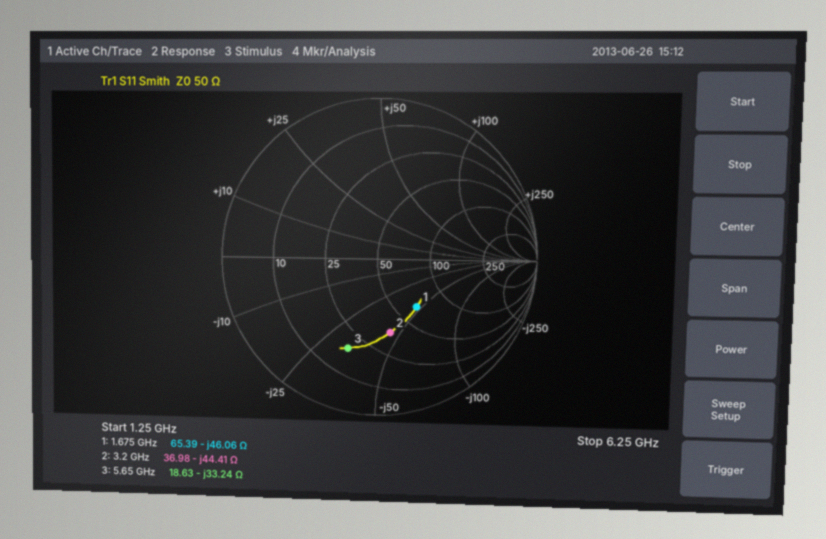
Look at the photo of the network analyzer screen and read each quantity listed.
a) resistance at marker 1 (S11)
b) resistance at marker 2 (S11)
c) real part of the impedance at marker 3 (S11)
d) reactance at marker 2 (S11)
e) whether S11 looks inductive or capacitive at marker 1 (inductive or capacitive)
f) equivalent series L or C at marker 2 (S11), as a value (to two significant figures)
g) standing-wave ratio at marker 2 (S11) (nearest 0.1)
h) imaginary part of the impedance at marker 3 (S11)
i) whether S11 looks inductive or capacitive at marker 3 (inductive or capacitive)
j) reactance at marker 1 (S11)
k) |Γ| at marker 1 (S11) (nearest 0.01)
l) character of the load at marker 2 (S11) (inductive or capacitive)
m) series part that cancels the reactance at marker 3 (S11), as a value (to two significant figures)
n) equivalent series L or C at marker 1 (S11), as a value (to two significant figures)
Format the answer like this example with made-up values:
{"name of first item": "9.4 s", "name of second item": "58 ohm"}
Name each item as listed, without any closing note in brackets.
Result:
{"resistance at marker 1": "65.39 Ω", "resistance at marker 2": "36.98 Ω", "real part of the impedance at marker 3": "18.63 Ω", "reactance at marker 2": "-44.41 Ω", "whether S11 looks inductive or capacitive at marker 1": "capacitive", "equivalent series L or C at marker 2 (S11), as a value": "1.1 pF", "standing-wave ratio at marker 2 (S11)": "2.8", "imaginary part of the impedance at marker 3": "-33.24 Ω", "whether S11 looks inductive or capacitive at marker 3": "capacitive", "reactance at marker 1": "-46.06 Ω", "|Γ| at marker 1 (S11)": "0.39", "character of the load at marker 2 (S11)": "capacitive", "series part that cancels the reactance at marker 3 (S11), as a value": "940 pH", "equivalent series L or C at marker 1 (S11), as a value": "2.1 pF"}
